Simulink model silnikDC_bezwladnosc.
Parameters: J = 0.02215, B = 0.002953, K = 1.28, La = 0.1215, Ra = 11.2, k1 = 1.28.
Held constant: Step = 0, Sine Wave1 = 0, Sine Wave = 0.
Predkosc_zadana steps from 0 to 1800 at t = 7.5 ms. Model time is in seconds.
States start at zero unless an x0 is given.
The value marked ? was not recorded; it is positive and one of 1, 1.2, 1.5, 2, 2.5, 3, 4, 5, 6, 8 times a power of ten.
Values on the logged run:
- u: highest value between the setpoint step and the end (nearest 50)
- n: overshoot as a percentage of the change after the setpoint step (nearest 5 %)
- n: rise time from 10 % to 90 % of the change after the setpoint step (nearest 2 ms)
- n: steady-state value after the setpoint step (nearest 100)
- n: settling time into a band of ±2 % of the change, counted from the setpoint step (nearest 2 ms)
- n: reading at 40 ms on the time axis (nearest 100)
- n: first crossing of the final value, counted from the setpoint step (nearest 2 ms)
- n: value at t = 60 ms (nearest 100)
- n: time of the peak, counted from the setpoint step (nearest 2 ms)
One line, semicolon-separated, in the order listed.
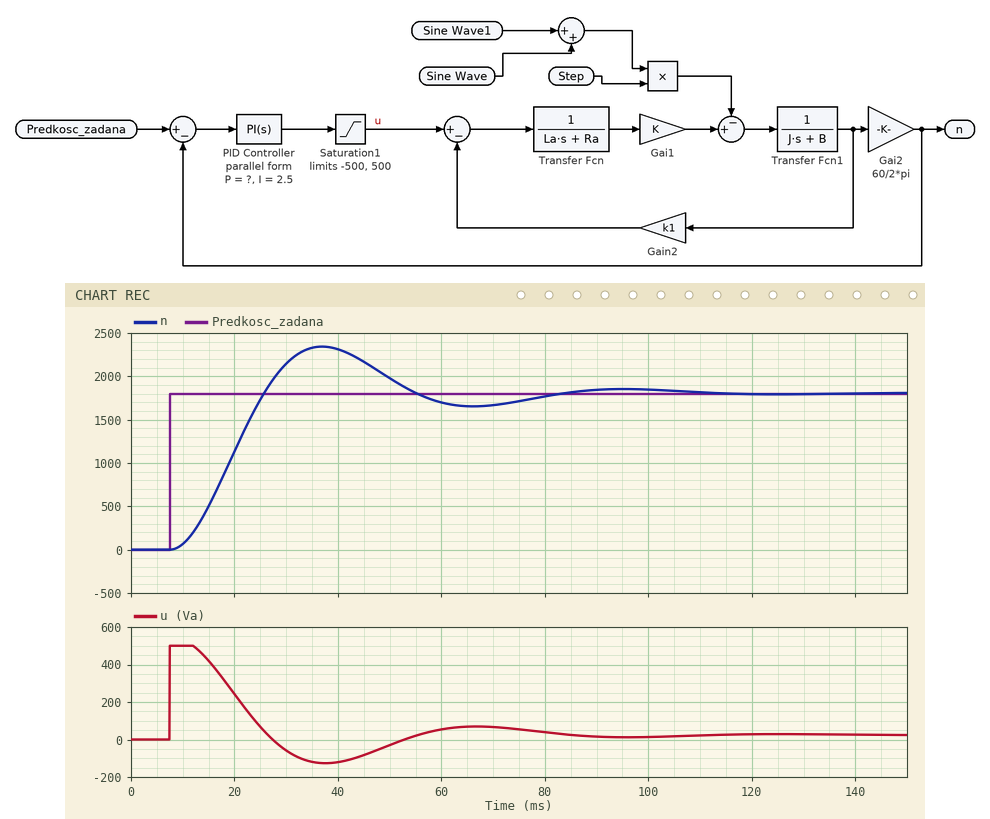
500; 30 %; 12 ms; 1800; 96 ms; 2300; 18 ms; 1700; 30 ms
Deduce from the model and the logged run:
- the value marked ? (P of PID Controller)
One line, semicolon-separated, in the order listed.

0.3
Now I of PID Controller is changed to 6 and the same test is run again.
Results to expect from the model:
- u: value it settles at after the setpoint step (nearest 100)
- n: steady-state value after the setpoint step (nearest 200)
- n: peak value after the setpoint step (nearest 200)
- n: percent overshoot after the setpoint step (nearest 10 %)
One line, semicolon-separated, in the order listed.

0; 1800; 2600; 40 %
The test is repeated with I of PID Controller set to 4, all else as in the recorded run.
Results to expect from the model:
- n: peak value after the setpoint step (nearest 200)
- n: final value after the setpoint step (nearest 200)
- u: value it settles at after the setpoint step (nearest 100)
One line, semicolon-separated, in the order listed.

2400; 1800; 0
